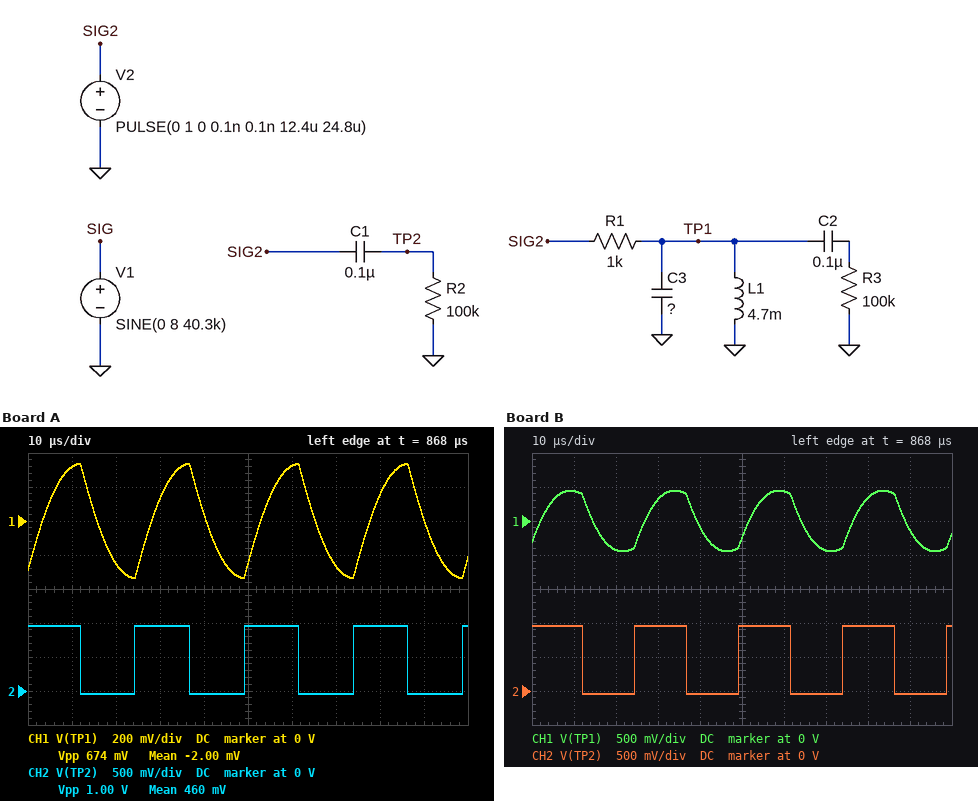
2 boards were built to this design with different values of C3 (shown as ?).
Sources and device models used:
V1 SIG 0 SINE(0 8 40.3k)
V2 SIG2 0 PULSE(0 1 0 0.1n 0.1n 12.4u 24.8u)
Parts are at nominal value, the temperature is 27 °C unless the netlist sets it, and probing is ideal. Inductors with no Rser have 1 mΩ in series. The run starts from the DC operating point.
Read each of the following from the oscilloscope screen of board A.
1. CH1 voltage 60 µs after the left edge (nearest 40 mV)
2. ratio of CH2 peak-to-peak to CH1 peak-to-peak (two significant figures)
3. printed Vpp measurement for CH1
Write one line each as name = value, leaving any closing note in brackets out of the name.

CH1 voltage 60 µs after the left edge = 320 mV
ratio of CH2 peak-to-peak to CH1 peak-to-peak = 1.5
printed Vpp measurement for CH1 = 674 mV
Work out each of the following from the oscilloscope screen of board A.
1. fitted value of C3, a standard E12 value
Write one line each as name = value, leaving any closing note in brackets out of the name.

fitted value of C3, a standard E12 value = 10 nF
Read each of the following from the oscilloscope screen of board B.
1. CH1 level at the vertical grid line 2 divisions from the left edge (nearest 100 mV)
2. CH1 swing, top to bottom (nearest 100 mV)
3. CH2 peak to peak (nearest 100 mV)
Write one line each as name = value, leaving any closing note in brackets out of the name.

CH1 level at the vertical grid line 2 divisions from the left edge = -400 mV
CH1 swing, top to bottom = 900 mV
CH2 peak to peak = 1.0 V
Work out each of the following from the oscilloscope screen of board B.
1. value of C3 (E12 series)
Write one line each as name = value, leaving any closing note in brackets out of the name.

value of C3 = 6.8 nF
